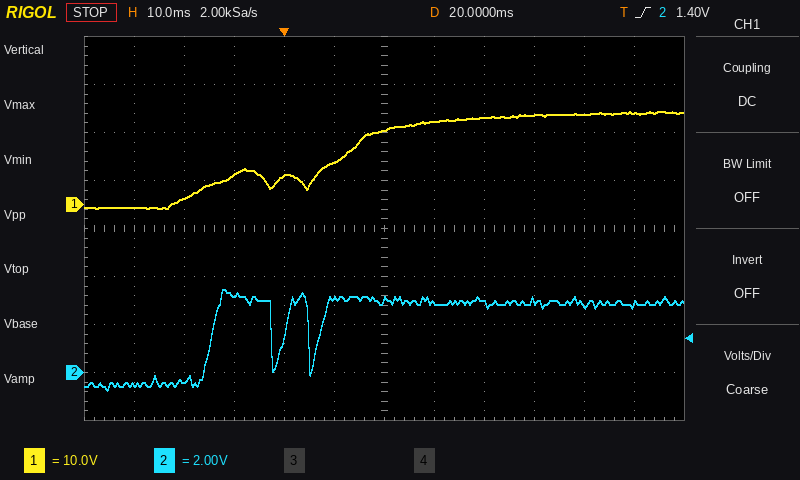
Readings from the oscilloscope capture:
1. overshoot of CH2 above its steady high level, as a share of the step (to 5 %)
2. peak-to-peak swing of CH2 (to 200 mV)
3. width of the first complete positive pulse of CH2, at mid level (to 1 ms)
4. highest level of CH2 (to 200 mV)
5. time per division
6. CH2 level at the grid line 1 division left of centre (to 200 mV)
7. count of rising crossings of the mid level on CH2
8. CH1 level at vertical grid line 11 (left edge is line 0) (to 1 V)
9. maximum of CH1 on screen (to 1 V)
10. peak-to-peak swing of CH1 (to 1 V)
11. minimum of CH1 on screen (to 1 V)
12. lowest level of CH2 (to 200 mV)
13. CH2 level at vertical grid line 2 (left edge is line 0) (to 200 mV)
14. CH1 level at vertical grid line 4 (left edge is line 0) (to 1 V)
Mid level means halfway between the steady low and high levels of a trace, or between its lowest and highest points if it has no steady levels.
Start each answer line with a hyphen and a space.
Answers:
- 15 %
- 4.2 V
- 12 ms
- 3.4 V
- 10 ms
- 3.0 V
- 3
- 19 V
- 19 V
- 20 V
- -1 V
- -800 mV
- -400 mV
- 6 V
